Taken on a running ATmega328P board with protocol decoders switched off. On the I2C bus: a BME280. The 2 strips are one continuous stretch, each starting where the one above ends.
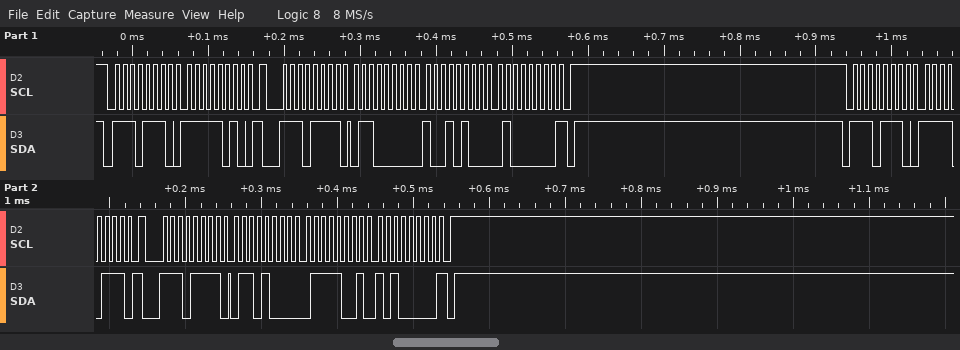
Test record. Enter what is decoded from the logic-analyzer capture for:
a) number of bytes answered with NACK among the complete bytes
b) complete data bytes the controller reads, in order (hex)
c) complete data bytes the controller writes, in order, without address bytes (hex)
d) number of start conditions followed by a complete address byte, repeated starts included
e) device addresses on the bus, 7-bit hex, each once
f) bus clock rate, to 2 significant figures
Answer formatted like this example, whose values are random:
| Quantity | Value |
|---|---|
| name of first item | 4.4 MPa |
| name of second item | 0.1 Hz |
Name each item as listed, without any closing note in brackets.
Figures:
| Quantity | Value |
|---|---|
| number of bytes answered with NACK among the complete bytes | 2 |
| complete data bytes the controller reads, in order | 60 94 40 68 79 A0 |
| complete data bytes the controller writes, in order, without address bytes | FA F7 |
| number of start conditions followed by a complete address byte, repeated starts included | 4 |
| device addresses on the bus, 7-bit hex, each once | 0x77 |
| bus clock rate, to 2 significant figures | 100 kHz |
